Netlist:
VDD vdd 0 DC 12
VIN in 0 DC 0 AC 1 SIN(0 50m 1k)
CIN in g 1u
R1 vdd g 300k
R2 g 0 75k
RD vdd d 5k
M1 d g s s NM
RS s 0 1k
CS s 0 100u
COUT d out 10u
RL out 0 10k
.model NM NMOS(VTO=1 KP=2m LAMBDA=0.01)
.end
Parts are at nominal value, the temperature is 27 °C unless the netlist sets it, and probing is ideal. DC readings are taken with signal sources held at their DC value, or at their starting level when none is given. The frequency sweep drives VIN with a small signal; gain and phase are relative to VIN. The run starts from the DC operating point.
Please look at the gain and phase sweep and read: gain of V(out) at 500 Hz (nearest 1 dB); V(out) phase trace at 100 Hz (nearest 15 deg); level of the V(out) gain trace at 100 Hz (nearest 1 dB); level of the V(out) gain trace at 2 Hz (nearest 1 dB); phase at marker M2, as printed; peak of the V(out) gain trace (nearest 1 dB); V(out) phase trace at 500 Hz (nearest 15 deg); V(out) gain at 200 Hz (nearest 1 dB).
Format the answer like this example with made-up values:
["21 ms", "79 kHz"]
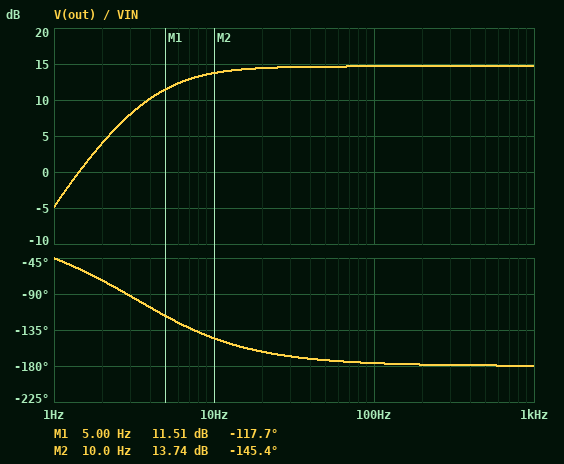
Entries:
["15 dB", "-180 deg", "15 dB", "4 dB", "-145.4 deg", "15 dB", "-180 deg", "15 dB"]
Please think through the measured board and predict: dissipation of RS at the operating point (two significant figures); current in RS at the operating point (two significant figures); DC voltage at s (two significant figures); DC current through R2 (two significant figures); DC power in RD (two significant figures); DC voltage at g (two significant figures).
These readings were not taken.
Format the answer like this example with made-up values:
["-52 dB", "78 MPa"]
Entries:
["400 µW", "630 µA", "630 mV", "32 µA", "2.0 mW", "2.4 V"]
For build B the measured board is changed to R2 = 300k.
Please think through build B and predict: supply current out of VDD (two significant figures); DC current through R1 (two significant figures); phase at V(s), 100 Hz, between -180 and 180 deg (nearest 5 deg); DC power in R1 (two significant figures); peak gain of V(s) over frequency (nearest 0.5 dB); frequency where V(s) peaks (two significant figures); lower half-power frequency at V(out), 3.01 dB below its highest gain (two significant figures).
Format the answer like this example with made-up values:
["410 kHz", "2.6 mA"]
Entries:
["2.0 mA", "20 µA", "-90 deg", "120 µW", "-36.5 dB", "1.7 Hz", "2.5 Hz"]
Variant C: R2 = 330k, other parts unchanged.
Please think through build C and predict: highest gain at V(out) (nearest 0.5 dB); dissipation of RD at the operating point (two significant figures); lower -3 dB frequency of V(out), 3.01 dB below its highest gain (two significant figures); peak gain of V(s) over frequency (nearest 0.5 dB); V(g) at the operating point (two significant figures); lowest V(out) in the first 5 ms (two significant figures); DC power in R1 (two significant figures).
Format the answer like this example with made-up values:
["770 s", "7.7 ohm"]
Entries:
["-20.5 dB", "19 mW", "2.5 Hz", "-38.0 dB", "6.3 V", "-4.7 mV", "110 µW"]
